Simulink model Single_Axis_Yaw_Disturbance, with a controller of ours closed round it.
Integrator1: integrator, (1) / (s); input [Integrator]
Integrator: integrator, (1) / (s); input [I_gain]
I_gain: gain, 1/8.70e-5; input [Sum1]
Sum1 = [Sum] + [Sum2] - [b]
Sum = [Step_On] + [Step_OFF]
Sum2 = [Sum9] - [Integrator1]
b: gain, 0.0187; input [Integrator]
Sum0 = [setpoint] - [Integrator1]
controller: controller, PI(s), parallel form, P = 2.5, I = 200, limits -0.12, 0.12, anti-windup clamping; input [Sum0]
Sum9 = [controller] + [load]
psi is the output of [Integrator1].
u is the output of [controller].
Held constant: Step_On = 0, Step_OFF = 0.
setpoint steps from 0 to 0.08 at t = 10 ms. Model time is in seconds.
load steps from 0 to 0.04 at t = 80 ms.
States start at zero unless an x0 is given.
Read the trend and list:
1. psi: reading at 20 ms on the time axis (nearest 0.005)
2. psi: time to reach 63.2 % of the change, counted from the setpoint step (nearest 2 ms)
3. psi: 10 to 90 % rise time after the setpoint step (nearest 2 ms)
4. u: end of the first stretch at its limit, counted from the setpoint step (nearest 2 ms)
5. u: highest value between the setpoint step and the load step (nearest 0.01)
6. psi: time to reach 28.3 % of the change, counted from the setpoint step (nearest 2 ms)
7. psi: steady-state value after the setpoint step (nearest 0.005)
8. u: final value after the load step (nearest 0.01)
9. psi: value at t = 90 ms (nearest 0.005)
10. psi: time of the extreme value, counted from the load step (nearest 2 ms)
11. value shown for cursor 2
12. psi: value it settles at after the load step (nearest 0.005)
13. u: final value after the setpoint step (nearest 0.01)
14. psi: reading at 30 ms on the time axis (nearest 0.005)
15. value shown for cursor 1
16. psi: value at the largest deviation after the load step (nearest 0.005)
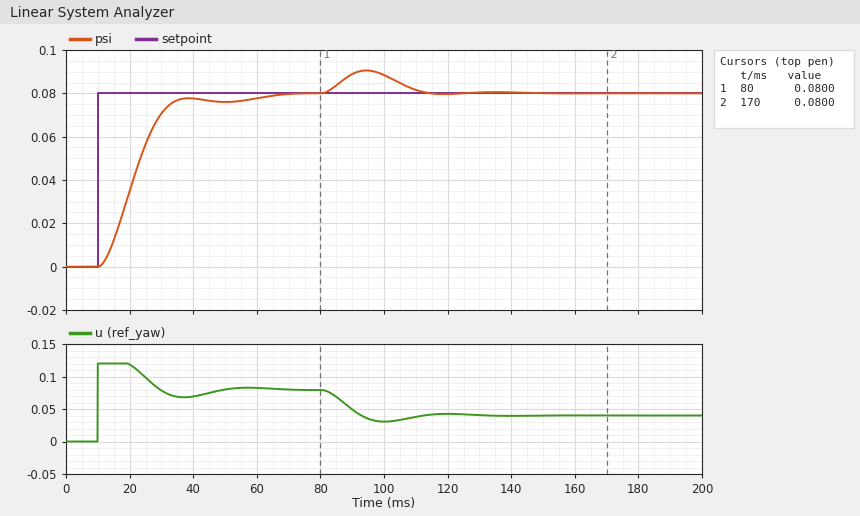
0.035
14 ms
16 ms
10 ms
0.12
8 ms
0.080
0.04
0.090
14 ms
0.0800
0.080
0.08
0.070
0.0800
0.090
